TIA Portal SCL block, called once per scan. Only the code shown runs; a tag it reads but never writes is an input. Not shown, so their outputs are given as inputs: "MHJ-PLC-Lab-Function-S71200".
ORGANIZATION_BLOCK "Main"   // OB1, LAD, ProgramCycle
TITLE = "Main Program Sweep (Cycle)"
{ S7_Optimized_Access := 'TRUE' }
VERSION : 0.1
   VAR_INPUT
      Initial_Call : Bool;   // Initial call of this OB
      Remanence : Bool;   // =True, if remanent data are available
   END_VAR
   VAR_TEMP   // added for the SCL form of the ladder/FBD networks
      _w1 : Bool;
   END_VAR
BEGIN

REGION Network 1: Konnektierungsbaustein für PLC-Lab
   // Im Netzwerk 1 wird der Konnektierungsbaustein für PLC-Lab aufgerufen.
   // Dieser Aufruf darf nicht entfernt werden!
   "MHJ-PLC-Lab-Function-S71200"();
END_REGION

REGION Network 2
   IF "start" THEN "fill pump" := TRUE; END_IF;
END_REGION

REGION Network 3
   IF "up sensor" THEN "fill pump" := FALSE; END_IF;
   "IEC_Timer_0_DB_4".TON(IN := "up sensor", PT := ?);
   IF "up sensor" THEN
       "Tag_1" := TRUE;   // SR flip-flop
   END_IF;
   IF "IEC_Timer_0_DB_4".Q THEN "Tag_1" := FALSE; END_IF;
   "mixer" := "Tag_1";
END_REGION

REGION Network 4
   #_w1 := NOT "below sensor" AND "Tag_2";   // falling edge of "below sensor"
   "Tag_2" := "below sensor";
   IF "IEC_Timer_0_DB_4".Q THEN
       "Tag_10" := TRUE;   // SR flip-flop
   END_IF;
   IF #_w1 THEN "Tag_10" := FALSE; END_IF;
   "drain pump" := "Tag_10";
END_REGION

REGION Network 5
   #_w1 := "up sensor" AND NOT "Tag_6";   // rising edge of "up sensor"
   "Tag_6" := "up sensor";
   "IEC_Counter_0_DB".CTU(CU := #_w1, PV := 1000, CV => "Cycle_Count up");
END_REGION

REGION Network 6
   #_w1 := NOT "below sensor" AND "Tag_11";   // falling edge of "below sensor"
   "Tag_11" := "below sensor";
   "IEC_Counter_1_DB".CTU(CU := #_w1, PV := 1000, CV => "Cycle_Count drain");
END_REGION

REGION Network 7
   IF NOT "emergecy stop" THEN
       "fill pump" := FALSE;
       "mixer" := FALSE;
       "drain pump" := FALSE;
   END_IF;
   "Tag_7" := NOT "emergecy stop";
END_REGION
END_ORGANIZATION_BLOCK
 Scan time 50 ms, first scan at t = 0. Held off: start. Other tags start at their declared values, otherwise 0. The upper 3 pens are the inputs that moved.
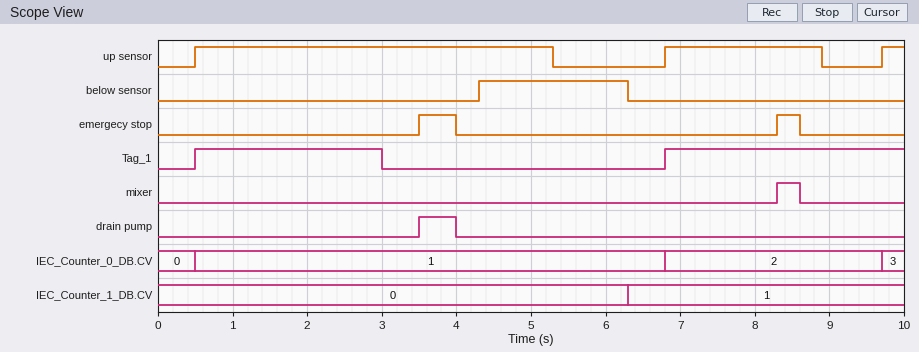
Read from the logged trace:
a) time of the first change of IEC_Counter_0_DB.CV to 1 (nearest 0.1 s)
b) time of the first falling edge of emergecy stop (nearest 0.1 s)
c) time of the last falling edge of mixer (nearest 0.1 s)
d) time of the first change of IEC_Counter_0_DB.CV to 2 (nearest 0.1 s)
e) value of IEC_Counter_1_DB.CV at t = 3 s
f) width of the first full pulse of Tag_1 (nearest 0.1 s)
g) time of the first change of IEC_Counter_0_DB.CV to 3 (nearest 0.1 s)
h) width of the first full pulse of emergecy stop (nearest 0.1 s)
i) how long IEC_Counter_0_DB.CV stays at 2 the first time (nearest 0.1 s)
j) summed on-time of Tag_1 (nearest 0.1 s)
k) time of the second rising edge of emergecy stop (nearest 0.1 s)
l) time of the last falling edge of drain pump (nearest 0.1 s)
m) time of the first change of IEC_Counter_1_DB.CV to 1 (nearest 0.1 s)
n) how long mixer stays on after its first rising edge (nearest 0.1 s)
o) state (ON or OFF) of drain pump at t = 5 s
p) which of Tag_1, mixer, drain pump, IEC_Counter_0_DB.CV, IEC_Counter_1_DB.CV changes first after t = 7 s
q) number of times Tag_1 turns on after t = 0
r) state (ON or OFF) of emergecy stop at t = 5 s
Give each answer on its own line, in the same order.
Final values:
0.5 s
4.0 s
8.6 s
6.8 s
0
2.5 s
9.7 s
0.5 s
2.9 s
5.7 s
8.3 s
4.0 s
6.3 s
0.3 s
OFF
mixer
2
OFF
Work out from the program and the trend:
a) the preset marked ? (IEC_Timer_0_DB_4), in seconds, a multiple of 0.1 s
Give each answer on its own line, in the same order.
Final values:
2.5 s
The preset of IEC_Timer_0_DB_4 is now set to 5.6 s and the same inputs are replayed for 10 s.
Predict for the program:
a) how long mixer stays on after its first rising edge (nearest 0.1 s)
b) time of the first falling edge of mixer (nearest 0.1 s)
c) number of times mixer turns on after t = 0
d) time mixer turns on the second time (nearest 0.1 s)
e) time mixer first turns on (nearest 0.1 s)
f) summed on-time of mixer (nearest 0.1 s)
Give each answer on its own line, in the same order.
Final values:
0.5 s
4.0 s
2
8.3 s
3.5 s
0.8 s
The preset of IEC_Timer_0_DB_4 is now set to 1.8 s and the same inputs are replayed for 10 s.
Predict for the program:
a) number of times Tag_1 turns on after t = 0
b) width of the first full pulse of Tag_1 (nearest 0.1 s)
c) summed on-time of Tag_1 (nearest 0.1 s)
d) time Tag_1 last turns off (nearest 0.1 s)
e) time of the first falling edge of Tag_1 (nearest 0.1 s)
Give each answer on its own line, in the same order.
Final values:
3
1.8 s
3.9 s
8.6 s
2.3 s
